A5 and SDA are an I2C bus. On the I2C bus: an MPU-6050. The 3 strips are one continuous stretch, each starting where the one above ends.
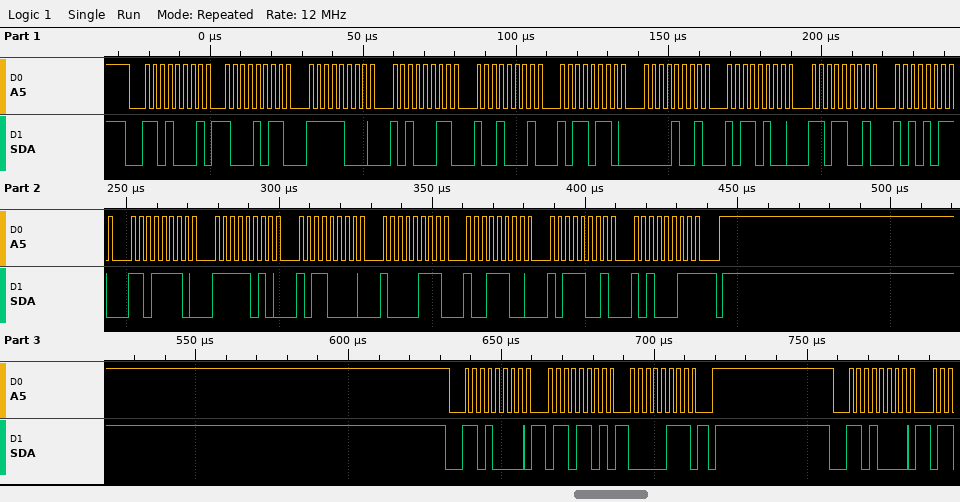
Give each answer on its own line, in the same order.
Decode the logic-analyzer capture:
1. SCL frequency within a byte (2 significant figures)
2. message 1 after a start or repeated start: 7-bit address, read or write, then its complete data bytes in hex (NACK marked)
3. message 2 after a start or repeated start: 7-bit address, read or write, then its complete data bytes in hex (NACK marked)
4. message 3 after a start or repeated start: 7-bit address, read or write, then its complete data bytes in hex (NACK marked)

400 kHz
0x68 read: 8B F8 A3 91 B6 09 B4 D9 AB DE FA B0 87 9C B9 A3 NACK
0x68 write: 6D 07
0x68 write
